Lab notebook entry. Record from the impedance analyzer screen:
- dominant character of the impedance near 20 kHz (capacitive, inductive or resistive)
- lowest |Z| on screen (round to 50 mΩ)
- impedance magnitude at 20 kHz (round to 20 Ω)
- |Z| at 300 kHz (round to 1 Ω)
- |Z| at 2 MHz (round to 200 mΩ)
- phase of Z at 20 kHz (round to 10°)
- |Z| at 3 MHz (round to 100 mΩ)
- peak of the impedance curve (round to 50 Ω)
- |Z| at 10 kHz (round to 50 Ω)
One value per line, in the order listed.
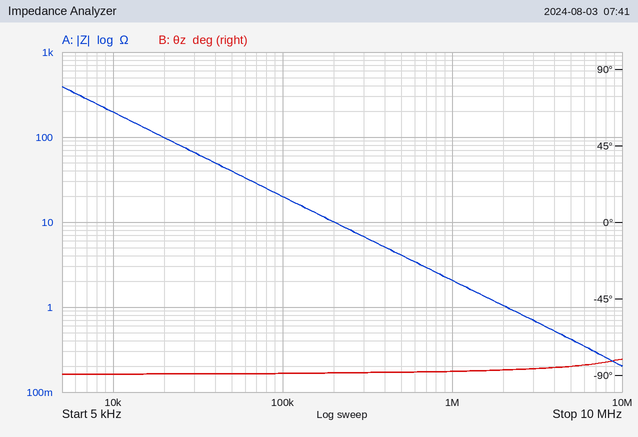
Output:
capacitive
200 mΩ
100 Ω
7 Ω
1.0 Ω
-90°
700 mΩ
400 Ω
200 Ω
